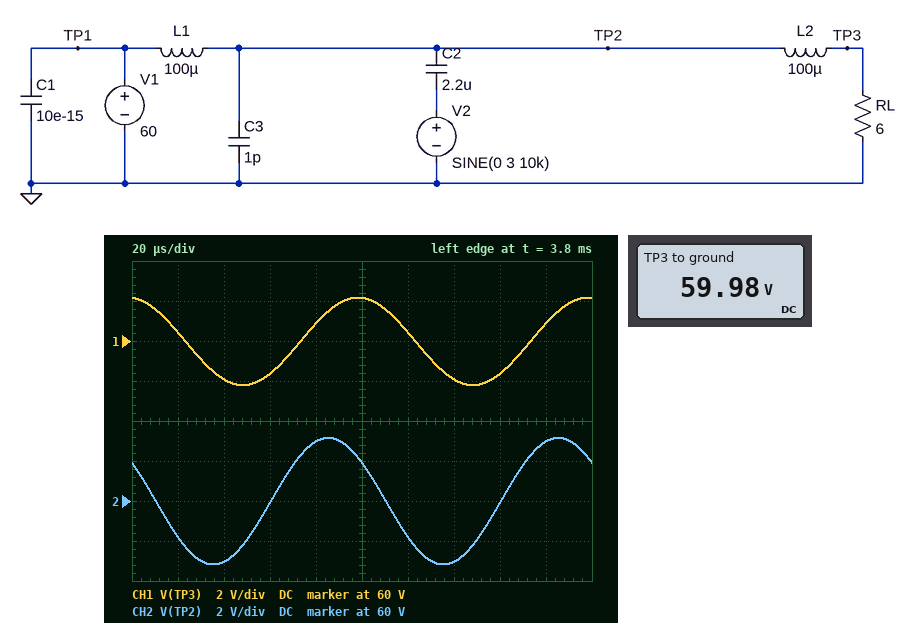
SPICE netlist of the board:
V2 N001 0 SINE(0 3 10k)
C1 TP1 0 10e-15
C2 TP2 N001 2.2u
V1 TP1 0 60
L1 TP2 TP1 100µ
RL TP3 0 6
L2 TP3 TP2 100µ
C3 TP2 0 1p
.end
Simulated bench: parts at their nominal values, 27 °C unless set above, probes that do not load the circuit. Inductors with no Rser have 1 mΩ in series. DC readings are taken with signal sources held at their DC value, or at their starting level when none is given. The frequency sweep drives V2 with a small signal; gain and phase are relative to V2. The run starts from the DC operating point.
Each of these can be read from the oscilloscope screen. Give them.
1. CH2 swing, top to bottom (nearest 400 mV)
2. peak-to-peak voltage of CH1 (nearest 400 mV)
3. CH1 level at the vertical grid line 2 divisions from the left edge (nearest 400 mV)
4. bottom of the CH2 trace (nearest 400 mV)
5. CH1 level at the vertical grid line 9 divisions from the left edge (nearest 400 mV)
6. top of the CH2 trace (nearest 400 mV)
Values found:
6.4 V
4.4 V
58.0 V
56.8 V
60.8 V
63.2 V
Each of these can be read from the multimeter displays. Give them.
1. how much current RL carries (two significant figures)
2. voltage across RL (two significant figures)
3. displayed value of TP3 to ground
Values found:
10 A
60 V
59.98 V
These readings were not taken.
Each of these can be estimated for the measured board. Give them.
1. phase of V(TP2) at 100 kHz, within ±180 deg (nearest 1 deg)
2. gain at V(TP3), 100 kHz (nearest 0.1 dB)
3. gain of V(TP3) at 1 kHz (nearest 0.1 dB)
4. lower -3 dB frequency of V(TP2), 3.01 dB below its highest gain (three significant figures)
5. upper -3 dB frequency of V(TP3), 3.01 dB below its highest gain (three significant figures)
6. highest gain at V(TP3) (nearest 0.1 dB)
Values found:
0 deg
-20.2 dB
-41.3 dB
12.8 kHz
16.8 kHz
6.5 dB
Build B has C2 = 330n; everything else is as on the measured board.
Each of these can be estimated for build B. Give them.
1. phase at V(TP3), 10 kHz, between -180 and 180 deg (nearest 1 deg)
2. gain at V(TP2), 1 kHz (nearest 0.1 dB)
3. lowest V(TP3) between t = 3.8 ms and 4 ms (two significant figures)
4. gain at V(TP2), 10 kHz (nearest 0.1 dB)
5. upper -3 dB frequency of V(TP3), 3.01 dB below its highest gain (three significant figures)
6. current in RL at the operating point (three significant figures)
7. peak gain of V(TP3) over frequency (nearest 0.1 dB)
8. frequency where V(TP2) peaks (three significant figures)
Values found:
114 deg
-57.8 dB
60 V
-21.1 dB
41.3 kHz
10.0 A
6.1 dB
39.0 kHz
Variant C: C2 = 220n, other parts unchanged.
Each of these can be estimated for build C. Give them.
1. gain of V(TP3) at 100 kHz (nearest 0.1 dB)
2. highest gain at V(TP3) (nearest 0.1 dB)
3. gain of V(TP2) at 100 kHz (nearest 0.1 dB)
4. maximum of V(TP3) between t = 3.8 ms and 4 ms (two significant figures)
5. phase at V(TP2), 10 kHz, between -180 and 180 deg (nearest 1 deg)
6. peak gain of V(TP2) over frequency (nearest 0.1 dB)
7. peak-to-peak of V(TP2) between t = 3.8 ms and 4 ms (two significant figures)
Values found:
-18.2 dB
6.1 dB
2.3 dB
60 V
161 deg
20.2 dB
340 mV
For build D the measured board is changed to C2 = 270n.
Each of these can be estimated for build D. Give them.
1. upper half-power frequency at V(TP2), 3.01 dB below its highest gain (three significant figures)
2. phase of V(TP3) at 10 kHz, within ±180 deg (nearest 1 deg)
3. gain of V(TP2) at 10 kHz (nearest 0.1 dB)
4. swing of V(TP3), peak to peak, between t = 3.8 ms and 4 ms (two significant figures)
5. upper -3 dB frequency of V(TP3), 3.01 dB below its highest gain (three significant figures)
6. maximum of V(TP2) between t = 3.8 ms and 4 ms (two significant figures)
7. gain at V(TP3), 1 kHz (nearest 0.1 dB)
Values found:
45.8 kHz
114 deg
-23.0 dB
290 mV
45.5 kHz
60 V
-59.6 dB
